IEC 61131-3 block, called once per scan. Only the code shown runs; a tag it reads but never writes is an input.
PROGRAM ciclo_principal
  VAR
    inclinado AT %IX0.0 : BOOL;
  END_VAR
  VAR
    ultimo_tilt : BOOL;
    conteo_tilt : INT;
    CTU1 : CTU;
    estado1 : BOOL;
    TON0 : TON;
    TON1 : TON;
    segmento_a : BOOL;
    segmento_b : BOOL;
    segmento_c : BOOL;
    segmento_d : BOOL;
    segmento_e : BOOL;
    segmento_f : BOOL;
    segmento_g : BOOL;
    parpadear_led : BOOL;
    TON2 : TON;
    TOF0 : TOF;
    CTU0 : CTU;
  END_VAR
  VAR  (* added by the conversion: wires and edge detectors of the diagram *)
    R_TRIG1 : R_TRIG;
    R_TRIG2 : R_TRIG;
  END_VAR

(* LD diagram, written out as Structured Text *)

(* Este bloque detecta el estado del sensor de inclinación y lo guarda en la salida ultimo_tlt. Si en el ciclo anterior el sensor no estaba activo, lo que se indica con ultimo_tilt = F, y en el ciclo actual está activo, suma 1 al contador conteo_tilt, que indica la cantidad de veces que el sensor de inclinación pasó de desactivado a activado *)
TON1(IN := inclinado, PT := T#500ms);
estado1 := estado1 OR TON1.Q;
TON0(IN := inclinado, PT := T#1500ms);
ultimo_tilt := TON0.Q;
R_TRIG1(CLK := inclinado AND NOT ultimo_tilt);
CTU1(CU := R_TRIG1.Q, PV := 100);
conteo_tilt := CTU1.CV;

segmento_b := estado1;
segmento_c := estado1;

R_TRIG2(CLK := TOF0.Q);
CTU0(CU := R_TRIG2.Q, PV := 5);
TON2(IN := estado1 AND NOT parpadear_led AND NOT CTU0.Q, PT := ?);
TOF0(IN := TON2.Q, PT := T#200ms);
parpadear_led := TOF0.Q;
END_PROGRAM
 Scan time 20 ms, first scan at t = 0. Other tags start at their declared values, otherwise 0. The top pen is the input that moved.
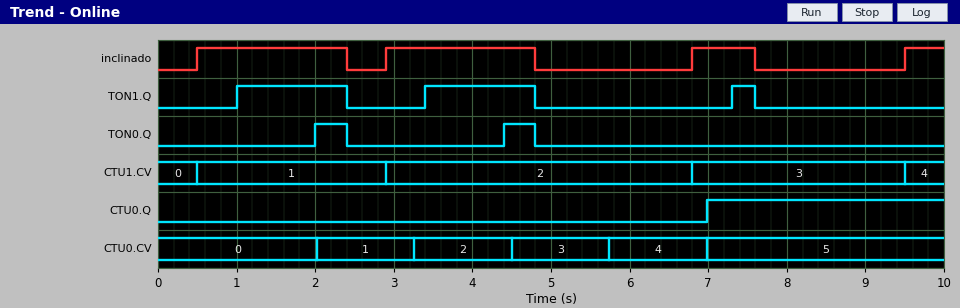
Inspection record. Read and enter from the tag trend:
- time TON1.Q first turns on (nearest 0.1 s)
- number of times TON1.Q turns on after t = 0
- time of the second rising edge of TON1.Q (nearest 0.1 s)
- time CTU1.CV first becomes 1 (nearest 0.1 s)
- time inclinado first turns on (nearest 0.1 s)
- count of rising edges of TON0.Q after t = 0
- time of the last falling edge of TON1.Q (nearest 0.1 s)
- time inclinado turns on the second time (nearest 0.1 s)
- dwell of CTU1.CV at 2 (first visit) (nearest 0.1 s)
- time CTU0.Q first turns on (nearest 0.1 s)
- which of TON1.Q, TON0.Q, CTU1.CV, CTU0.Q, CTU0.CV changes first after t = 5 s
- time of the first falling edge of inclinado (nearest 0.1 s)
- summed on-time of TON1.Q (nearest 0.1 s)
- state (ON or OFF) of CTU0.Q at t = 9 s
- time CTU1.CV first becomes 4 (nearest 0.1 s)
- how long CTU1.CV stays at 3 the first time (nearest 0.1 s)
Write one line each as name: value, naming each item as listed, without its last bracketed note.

time TON1.Q first turns on: 1.0 s
number of times TON1.Q turns on after t = 0: 3
time of the second rising edge of TON1.Q: 3.4 s
time CTU1.CV first becomes 1: 0.5 s
time inclinado first turns on: 0.5 s
count of rising edges of TON0.Q after t = 0: 2
time of the last falling edge of TON1.Q: 7.6 s
time inclinado turns on the second time: 2.9 s
dwell of CTU1.CV at 2 (first visit): 3.9 s
time CTU0.Q first turns on: 7.0 s
which of TON1.Q, TON0.Q, CTU1.CV, CTU0.Q, CTU0.CV changes first after t = 5 s: CTU0.CV
time of the first falling edge of inclinado: 2.4 s
summed on-time of TON1.Q: 3.1 s
state (ON or OFF) of CTU0.Q at t = 9 s: ON
time CTU1.CV first becomes 4: 9.5 s
how long CTU1.CV stays at 3 the first time: 2.7 s
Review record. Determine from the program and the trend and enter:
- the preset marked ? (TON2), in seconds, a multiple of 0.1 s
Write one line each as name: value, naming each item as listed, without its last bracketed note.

the preset marked ? (TON2), in seconds, a multiple of 0.1 s: 1.0 s
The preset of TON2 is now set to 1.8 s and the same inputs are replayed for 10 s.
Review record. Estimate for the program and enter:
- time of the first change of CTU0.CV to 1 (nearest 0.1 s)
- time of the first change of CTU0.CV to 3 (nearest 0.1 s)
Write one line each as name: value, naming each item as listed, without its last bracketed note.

time of the first change of CTU0.CV to 1: 2.8 s
time of the first change of CTU0.CV to 3: 6.9 s
